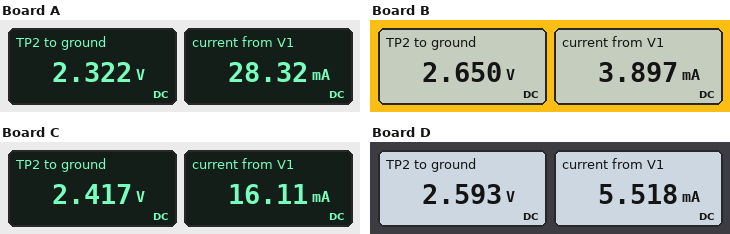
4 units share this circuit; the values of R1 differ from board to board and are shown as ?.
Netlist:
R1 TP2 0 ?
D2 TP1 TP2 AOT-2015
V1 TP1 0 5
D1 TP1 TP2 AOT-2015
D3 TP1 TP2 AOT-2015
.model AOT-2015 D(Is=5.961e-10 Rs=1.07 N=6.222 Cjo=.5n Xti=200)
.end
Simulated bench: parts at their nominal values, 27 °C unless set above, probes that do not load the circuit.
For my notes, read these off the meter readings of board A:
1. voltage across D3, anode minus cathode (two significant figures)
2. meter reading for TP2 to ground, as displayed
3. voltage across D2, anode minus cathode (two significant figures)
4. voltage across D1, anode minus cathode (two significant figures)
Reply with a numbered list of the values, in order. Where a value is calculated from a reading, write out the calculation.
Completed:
1. 5 V - 2.322 V = 2.7 V
2. 2.322 V
3. 5 V - 2.322 V = 2.7 V
4. 5 V - 2.322 V = 2.7 V
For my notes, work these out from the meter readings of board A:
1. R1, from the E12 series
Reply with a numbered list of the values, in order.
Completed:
1. 82 Ω
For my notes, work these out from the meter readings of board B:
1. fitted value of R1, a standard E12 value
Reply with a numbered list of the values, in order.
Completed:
1. 680 Ω
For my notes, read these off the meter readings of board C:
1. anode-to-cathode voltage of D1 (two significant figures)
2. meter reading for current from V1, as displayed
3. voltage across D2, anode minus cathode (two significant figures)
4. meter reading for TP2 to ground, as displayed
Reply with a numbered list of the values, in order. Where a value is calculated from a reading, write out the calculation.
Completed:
1. 5 V - 2.417 V = 2.6 V
2. 16.11 mA
3. 5 V - 2.417 V = 2.6 V
4. 2.417 V
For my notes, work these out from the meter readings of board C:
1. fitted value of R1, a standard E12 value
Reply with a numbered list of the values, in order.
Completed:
1. 150 Ω
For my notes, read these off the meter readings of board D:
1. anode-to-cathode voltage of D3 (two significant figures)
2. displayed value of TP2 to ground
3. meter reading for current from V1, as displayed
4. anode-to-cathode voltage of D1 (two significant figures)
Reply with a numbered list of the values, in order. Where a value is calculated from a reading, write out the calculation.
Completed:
1. 5 V - 2.593 V = 2.4 V
2. 2.593 V
3. 5.518 mA
4. 5 V - 2.593 V = 2.4 V
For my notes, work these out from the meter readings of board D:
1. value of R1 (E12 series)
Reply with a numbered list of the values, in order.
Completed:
1. 470 Ω
